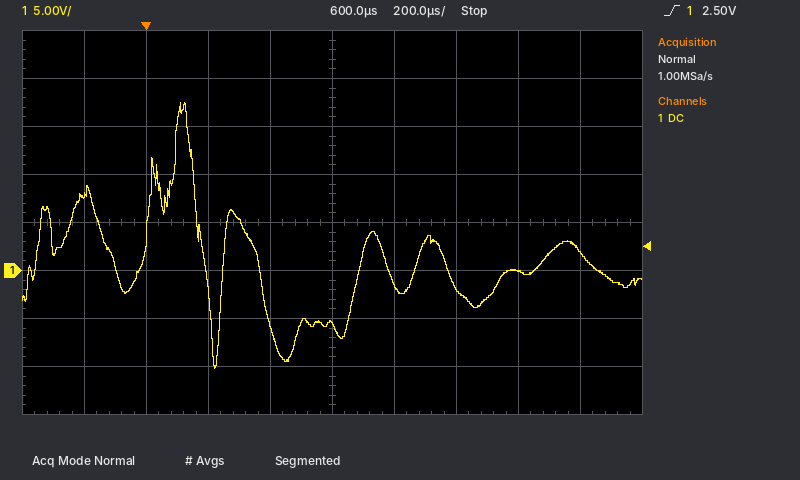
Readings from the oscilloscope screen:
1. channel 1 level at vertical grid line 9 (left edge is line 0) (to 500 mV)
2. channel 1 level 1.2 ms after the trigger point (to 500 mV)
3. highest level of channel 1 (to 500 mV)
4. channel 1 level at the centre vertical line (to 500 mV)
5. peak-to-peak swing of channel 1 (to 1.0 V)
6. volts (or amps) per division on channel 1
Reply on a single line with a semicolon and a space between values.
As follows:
2.0 V; 0.0 V; 17.5 V; -5.5 V; 28.0 V; 5 V
